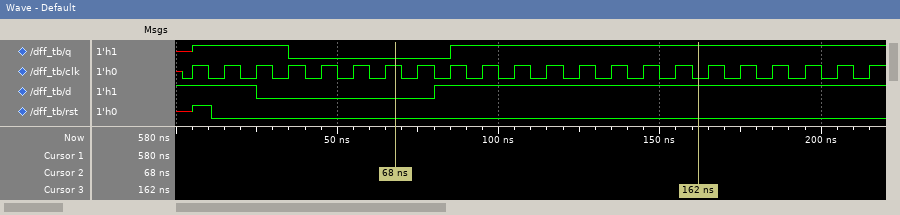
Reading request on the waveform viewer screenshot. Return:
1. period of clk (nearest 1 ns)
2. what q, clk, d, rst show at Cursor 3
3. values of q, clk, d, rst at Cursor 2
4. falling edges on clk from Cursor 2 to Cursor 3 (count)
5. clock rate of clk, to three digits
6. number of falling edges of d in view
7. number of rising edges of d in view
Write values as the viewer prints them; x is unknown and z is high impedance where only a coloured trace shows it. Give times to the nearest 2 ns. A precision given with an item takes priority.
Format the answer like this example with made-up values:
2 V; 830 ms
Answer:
10 ns; q=1, clk=0, d=1, rst=0; q=0, clk=1, d=0, rst=0; 10; 100 MHz; 1; 1
